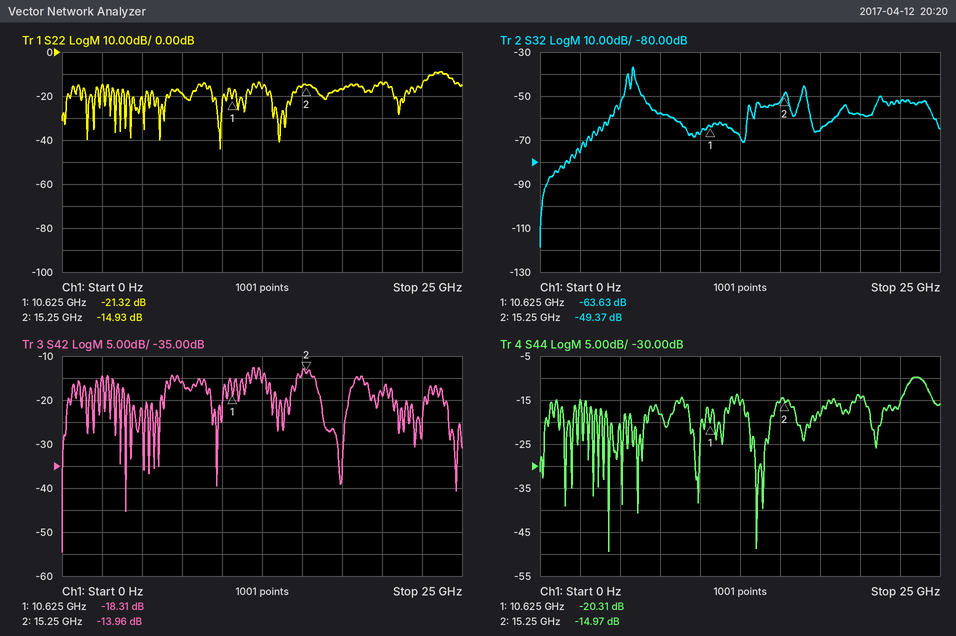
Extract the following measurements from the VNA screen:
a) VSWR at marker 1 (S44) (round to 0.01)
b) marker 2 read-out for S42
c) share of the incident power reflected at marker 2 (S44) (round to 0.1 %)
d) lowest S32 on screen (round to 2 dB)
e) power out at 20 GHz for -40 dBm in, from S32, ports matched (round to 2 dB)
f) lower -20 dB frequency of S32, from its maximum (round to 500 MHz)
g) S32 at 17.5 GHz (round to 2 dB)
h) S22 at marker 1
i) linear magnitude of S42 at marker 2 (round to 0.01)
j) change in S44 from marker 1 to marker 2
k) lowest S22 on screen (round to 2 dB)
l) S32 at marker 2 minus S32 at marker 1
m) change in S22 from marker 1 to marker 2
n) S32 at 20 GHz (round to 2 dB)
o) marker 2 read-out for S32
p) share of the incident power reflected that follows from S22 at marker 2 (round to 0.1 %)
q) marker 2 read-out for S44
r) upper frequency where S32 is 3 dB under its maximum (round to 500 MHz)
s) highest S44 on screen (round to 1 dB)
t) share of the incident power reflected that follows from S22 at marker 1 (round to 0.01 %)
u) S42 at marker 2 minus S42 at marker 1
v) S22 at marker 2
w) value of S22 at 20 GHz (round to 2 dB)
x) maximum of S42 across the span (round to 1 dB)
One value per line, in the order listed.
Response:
1.21
-13.96 dB
3.2 %
-118 dB
-98 dBm
4.5 GHz
-66 dB
-21.32 dB
0.20
5.34 dB
-44 dB
14.26 dB
6.39 dB
-58 dB
-49.37 dB
3.2 %
-14.97 dB
6.0 GHz
-10 dB
0.74 %
4.35 dB
-14.93 dB
-14 dB
-13 dB
